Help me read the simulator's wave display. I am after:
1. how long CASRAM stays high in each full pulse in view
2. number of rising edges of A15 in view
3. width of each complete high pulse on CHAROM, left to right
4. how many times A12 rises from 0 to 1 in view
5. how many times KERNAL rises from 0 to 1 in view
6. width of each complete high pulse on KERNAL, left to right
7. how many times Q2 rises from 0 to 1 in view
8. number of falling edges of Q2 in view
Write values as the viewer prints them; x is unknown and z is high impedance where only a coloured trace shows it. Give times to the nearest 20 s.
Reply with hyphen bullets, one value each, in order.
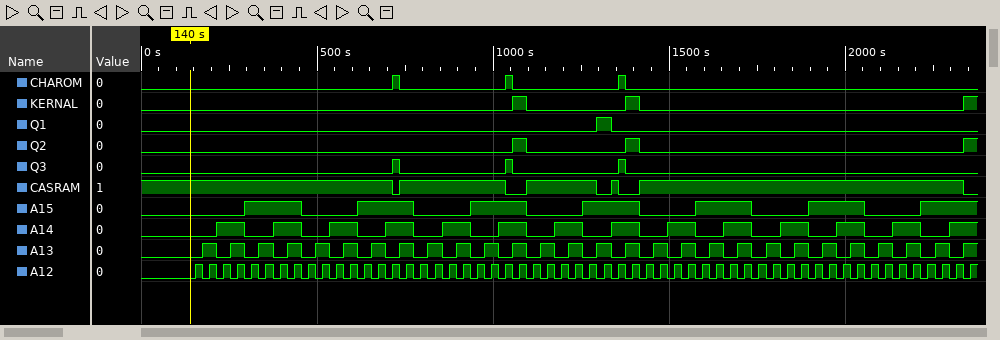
- 300 s, 200 s, 20 s, 920 s
- 7
- 20 s, 20 s, 20 s
- 56
- 3
- 40 s, 40 s
- 3
- 2
